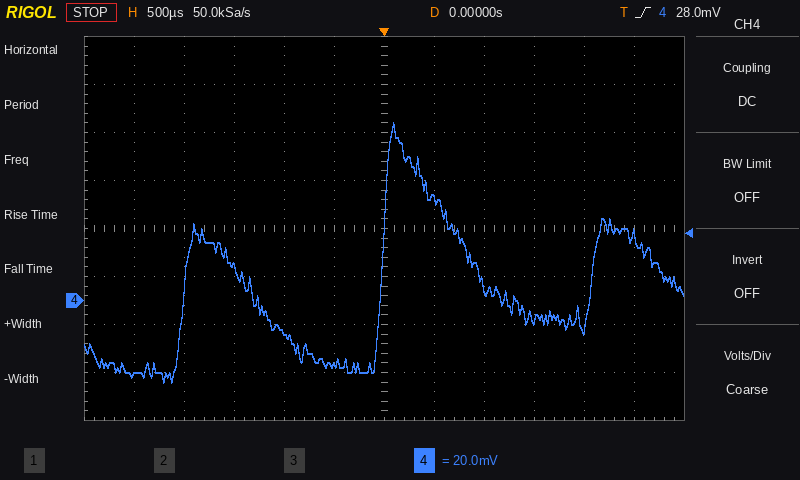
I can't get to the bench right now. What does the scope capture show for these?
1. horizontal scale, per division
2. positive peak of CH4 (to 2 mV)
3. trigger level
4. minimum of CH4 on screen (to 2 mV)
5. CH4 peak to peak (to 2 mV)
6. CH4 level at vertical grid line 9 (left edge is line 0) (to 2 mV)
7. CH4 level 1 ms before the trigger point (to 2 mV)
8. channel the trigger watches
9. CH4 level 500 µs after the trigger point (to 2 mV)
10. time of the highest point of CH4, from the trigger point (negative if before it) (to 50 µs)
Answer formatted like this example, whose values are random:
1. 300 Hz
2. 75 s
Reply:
1. 500 µs
2. 74 mV
3. 28.0 mV
4. -34 mV
5. 108 mV
6. -8 mV
7. -14 mV
8. CH4
9. 42 mV
10. +100 µs
